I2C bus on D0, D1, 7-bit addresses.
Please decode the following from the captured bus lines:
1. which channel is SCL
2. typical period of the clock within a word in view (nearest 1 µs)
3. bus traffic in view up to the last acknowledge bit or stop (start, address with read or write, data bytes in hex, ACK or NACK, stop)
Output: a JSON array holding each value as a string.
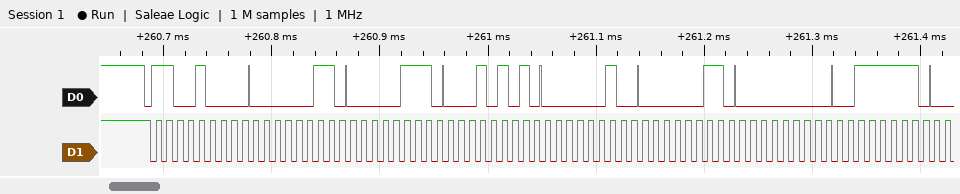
["D1", "10 µs", "start, address 64 write ACK, 03 ACK, 07 ACK, 15 ACK, 02 ACK, 03 ACK, 00 ACK, 3F ACK"]
